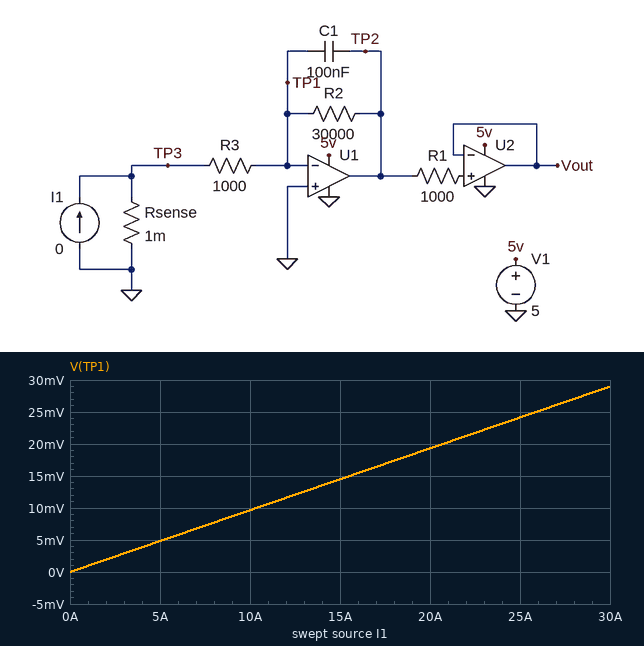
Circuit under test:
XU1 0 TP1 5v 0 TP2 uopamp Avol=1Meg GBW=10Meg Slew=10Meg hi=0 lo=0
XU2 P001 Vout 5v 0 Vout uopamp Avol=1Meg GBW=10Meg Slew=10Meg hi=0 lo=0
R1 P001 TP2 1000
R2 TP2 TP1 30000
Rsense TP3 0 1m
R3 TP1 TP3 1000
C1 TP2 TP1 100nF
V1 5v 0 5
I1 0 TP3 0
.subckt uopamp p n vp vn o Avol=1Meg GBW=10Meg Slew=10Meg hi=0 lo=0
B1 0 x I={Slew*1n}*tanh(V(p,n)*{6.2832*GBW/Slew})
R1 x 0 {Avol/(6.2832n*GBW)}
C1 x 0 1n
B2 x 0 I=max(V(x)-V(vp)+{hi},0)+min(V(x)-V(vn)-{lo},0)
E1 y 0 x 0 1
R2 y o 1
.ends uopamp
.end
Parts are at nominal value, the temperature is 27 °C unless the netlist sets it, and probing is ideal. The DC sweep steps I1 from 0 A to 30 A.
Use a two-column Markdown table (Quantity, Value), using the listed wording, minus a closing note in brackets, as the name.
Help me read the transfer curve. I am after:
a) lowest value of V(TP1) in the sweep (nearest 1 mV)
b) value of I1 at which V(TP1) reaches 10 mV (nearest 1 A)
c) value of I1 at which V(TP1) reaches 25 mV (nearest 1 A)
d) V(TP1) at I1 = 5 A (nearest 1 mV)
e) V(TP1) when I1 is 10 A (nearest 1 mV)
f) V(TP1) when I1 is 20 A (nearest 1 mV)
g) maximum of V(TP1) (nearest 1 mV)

| Quantity | Value |
|---|---|
| lowest value of V(TP1) in the sweep | 0 V |
| value of I1 at which V(TP1) reaches 10 mV | 10 A |
| value of I1 at which V(TP1) reaches 25 mV | 26 A |
| V(TP1) at I1 = 5 A | 5 mV |
| V(TP1) when I1 is 10 A | 10 mV |
| V(TP1) when I1 is 20 A | 19 mV |
| maximum of V(TP1) | 29 mV |
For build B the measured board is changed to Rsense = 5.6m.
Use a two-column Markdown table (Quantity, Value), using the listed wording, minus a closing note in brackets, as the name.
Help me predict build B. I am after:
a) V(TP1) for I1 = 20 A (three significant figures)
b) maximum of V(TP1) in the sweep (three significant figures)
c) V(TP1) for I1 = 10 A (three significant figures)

| Quantity | Value |
|---|---|
| V(TP1) for I1 = 20 A | 108 mV |
| maximum of V(TP1) in the sweep | 162 mV |
| V(TP1) for I1 = 10 A | 54.1 mV |
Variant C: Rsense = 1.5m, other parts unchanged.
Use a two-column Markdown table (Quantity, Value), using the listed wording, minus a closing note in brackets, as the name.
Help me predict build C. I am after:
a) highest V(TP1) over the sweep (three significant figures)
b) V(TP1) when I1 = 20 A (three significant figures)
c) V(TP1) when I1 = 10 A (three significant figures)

| Quantity | Value |
|---|---|
| highest V(TP1) over the sweep | 43.5 mV |
| V(TP1) when I1 = 20 A | 29.0 mV |
| V(TP1) when I1 = 10 A | 14.5 mV |
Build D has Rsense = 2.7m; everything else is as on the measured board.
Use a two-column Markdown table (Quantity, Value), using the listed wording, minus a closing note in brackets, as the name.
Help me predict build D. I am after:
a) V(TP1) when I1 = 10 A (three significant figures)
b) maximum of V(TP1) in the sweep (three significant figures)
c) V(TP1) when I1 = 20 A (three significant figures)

| Quantity | Value |
|---|---|
| V(TP1) when I1 = 10 A | 26.1 mV |
| maximum of V(TP1) in the sweep | 78.2 mV |
| V(TP1) when I1 = 20 A | 52.2 mV |
